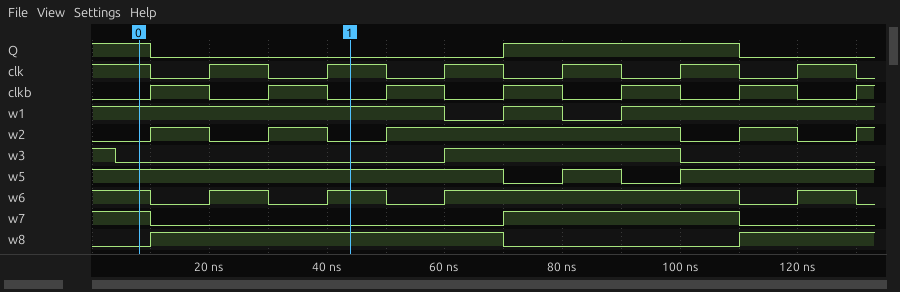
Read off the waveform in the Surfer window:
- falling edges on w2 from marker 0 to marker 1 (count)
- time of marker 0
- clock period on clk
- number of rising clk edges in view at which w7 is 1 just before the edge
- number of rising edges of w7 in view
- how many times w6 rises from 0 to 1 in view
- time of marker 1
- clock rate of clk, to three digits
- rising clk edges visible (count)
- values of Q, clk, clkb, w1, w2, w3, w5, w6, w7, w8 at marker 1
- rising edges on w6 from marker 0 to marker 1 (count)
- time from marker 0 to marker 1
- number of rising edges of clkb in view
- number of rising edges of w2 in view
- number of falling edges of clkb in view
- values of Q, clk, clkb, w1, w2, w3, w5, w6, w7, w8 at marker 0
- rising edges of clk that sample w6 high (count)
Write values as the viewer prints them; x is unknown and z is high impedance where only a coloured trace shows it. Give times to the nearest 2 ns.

2
8 ns
20 ns
2
1
4
44 ns
50.0 MHz
6
Q=0, clk=1, clkb=0, w1=1, w2=0, w3=0, w5=1, w6=1, w7=0, w8=1
2
36 ns
7
5
6
Q=1, clk=1, clkb=0, w1=1, w2=0, w3=0, w5=1, w6=1, w7=1, w8=0
2
